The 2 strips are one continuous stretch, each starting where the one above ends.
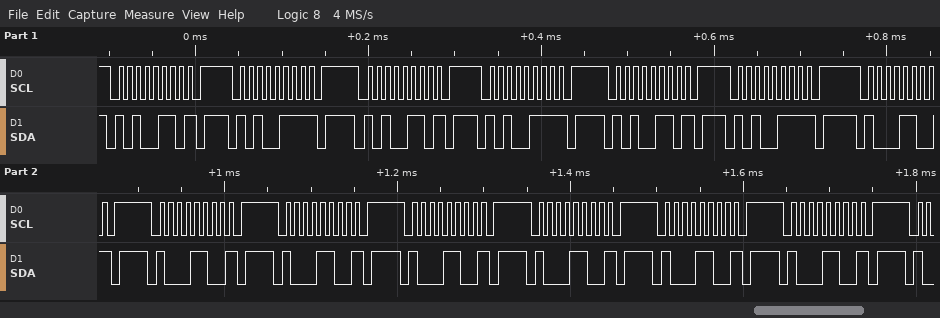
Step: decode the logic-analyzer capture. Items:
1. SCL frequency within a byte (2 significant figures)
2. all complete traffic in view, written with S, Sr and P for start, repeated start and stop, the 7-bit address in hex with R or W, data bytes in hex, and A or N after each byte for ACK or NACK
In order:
100 kHz
S 53W N P S 53R N P S 53W N P S 53R N P S 53W N P S 53R N P S 46W N P S 46W N P S 46W N P S 46W N P S 46W N P S 46W N P S 46W N P
